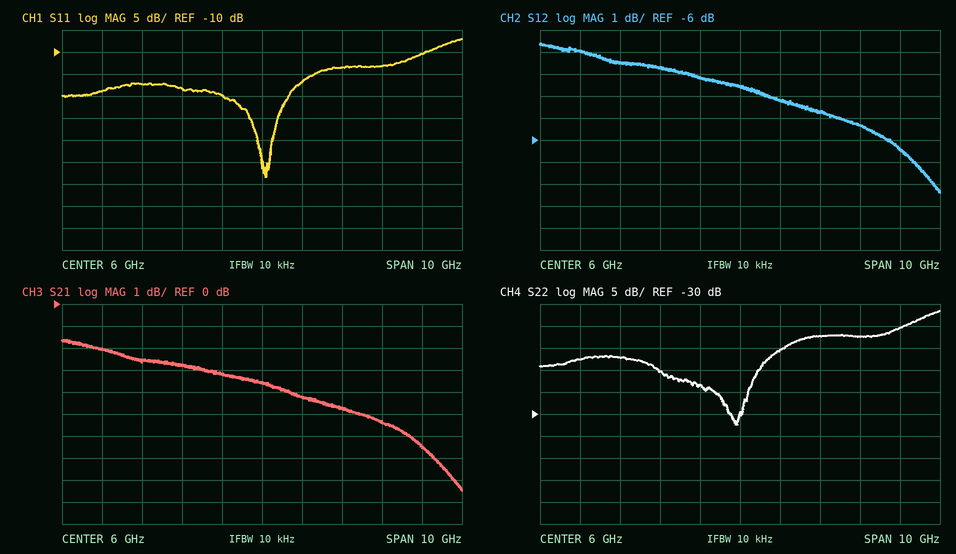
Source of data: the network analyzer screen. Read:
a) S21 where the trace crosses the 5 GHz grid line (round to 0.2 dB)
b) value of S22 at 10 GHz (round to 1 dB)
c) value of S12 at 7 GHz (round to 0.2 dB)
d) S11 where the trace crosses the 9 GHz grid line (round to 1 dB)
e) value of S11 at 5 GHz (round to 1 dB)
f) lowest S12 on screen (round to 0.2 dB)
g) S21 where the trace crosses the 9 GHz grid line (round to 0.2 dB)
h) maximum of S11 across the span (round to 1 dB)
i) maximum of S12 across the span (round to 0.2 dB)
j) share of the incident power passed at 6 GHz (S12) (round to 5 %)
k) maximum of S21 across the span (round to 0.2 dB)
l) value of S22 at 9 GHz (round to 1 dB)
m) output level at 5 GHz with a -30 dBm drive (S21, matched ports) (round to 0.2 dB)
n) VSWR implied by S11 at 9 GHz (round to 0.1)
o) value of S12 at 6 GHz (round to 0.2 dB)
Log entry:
-3.2 dB
-10 dB
-4.2 dB
-13 dB
-20 dB
-8.4 dB
-5.4 dB
-7 dB
-1.6 dB
45 %
-1.6 dB
-12 dB
-33.2 dBm
1.6
-3.6 dB
